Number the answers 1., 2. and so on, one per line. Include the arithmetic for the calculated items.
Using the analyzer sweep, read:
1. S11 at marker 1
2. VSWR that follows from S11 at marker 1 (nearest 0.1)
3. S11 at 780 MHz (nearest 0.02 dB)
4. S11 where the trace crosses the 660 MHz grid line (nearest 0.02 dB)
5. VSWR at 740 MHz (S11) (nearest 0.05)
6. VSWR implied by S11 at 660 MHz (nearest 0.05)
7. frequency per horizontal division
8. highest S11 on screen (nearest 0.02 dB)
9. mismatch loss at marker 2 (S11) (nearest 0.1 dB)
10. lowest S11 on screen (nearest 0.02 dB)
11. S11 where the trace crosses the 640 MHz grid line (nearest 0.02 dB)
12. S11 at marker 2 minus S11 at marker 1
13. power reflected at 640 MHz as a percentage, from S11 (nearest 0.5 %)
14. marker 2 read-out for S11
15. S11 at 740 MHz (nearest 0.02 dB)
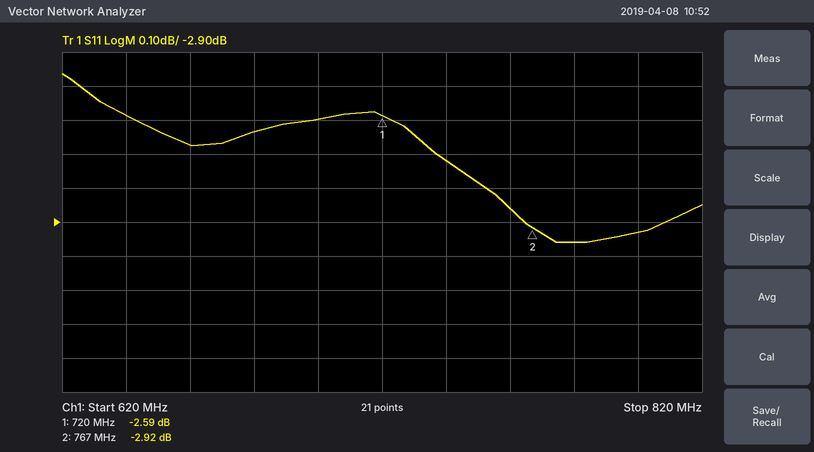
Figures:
1. -2.59 dB
2. (1 + 0.7422)/(1 − 0.7422) ≈ 6.8
3. -2.96 dB
4. -2.68 dB
5. |Γ| = 10^(-2.72/20) = 0.7311; VSWR = (1 + 0.7311)/(1 − 0.7311) ≈ 6.44, so 6.45 to the nearest 0.05
6. |Γ| = 10^(-2.68/20) = 0.7345; VSWR = (1 + 0.7345)/(1 − 0.7345) ≈ 6.53, so 6.55 to the nearest 0.05
7. 20 MHz
8. -2.46 dB
9. −10 log10(1 − 10^(-2.92/10)) ≈ 3.1 dB
10. -2.96 dB
11. -2.58 dB
12. -2.92 − (-2.59) = -0.33 dB
13. 10^(-2.58/10) ≈ 55.2 %, so 55.0 % to the nearest 0.5 %
14. -2.92 dB
15. -2.72 dB
